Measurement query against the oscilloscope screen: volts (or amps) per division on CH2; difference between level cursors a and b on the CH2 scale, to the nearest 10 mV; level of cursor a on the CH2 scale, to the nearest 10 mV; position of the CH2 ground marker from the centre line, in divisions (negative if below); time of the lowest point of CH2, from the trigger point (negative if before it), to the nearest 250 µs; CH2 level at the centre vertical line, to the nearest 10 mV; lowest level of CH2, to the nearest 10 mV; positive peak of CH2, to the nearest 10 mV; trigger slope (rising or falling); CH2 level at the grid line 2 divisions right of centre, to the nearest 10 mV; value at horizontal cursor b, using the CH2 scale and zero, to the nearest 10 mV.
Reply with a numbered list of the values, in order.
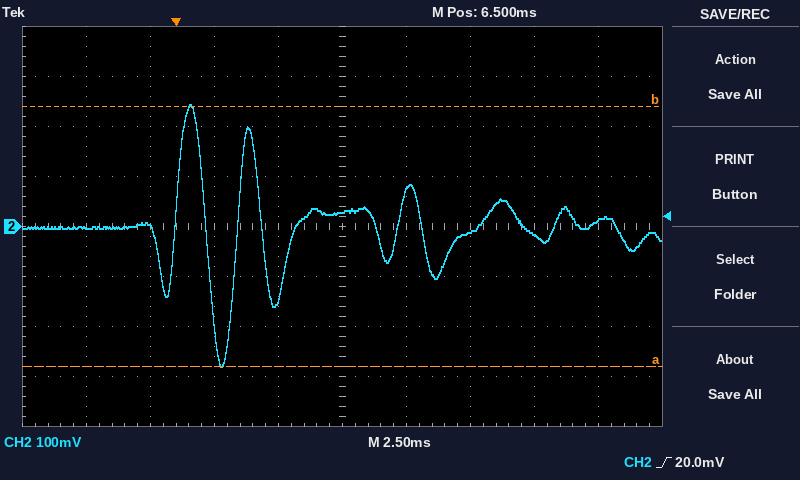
1. 100 mV
2. 520 mV
3. -280 mV
4. 0.0 div
5. +1.75 ms
6. 30 mV
7. -280 mV
8. 240 mV
9. rising
10. -10 mV
11. 240 mV
